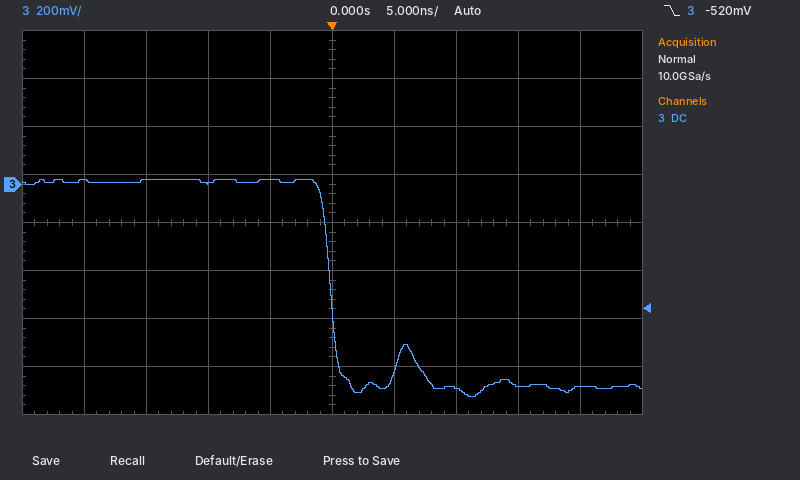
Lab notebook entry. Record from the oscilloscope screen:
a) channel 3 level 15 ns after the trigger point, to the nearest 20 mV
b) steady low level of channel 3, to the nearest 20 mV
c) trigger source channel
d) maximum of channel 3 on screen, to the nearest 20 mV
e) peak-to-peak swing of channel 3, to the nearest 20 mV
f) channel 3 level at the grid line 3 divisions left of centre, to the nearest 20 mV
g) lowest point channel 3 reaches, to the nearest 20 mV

-840 mV
-840 mV
channel 3
20 mV
900 mV
20 mV
-880 mV
